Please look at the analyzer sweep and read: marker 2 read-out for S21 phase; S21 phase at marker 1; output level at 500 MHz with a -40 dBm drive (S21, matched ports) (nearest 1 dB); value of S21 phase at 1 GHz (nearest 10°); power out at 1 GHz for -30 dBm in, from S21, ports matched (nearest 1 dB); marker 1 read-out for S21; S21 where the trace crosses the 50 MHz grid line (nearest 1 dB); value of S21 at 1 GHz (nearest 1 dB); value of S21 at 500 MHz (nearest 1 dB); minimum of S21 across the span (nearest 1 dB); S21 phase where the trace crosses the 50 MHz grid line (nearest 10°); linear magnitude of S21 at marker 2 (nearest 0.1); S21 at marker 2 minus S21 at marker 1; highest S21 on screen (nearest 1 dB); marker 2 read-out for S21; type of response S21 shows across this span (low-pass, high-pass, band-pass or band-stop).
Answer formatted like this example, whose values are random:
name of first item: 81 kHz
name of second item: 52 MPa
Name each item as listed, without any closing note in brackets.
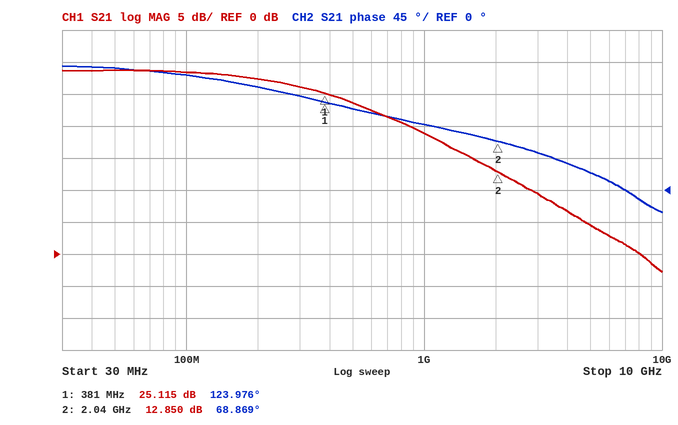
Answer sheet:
marker 2 read-out for S21 phase: 68.869°
S21 phase at marker 1: 123.976°
output level at 500 MHz with a -40 dBm drive (S21, matched ports): -16 dBm
value of S21 phase at 1 GHz: 90°
power out at 1 GHz for -30 dBm in, from S21, ports matched: -11 dBm
marker 1 read-out for S21: 25.115 dB
S21 where the trace crosses the 50 MHz grid line: 29 dB
value of S21 at 1 GHz: 19 dB
value of S21 at 500 MHz: 24 dB
minimum of S21 across the span: -3 dB
S21 phase where the trace crosses the 50 MHz grid line: 170°
linear magnitude of S21 at marker 2: 4.4
S21 at marker 2 minus S21 at marker 1: -12.265 dB
highest S21 on screen: 29 dB
marker 2 read-out for S21: 12.850 dB
type of response S21 shows across this span: low-pass
